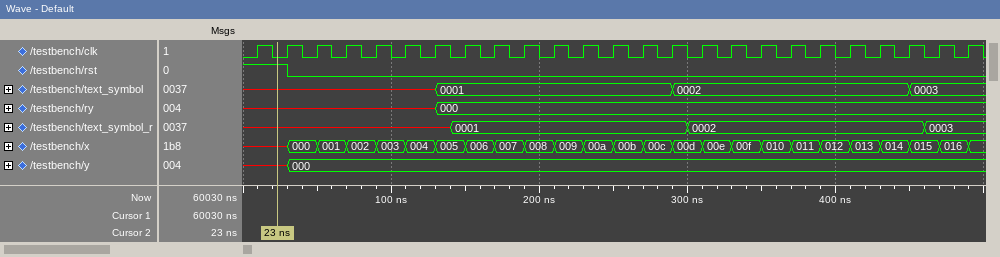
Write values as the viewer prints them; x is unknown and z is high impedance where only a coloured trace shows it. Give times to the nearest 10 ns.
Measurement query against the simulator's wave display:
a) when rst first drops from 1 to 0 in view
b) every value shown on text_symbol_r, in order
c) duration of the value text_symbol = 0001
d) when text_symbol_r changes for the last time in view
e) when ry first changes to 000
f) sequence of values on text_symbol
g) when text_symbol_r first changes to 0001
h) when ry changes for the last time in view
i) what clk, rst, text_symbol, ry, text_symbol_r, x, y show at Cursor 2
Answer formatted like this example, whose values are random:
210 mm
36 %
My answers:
30 ns
x, 0001, 0002, 0003
160 ns
460 ns
130 ns
x, 0001, 0002, 0003
140 ns
130 ns
clk=0, rst=1, text_symbol=x, ry=x, text_symbol_r=x, x=x, y=x
